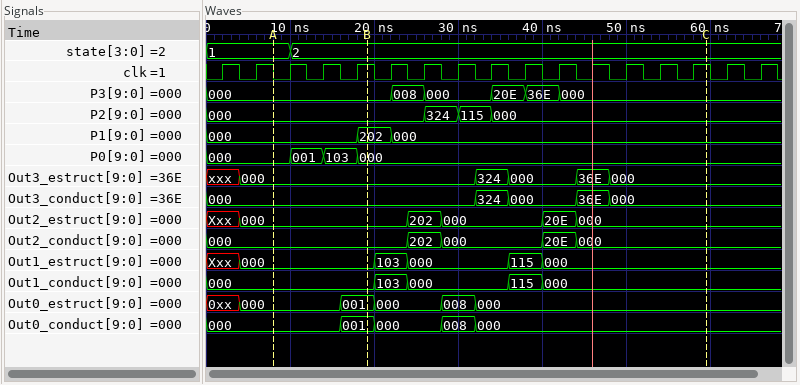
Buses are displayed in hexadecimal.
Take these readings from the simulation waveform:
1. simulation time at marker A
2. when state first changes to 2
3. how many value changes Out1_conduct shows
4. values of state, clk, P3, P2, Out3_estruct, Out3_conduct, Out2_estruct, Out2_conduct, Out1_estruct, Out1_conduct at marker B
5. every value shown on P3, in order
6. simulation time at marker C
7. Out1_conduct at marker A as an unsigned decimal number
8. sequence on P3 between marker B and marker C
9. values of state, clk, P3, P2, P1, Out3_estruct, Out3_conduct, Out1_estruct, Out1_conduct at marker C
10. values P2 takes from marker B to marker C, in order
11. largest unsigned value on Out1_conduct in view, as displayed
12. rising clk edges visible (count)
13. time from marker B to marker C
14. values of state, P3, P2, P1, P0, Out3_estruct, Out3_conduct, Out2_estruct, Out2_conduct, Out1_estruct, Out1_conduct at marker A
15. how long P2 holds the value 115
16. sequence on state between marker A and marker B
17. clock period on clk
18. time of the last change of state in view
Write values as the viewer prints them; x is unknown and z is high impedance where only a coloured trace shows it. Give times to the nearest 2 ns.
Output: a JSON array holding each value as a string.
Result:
["8 ns", "10 ns", "4", "state=2, clk=1, P3=000, P2=000, Out3_estruct=000, Out3_conduct=000, Out2_estruct=000, Out2_conduct=000, Out1_estruct=000, Out1_conduct=000", "000, 008, 000, 20E, 36E, 000", "60 ns", "0", "000, 008, 000, 20E, 36E, 000", "state=2, clk=1, P3=000, P2=000, P1=000, Out3_estruct=000, Out3_conduct=000, Out1_estruct=000, Out1_conduct=000", "000, 324, 115, 000", "115", "17", "40 ns", "state=1, P3=000, P2=000, P1=000, P0=000, Out3_estruct=000, Out3_conduct=000, Out2_estruct=000, Out2_conduct=000, Out1_estruct=000, Out1_conduct=000", "4 ns", "1, 2", "4 ns", "10 ns"]
